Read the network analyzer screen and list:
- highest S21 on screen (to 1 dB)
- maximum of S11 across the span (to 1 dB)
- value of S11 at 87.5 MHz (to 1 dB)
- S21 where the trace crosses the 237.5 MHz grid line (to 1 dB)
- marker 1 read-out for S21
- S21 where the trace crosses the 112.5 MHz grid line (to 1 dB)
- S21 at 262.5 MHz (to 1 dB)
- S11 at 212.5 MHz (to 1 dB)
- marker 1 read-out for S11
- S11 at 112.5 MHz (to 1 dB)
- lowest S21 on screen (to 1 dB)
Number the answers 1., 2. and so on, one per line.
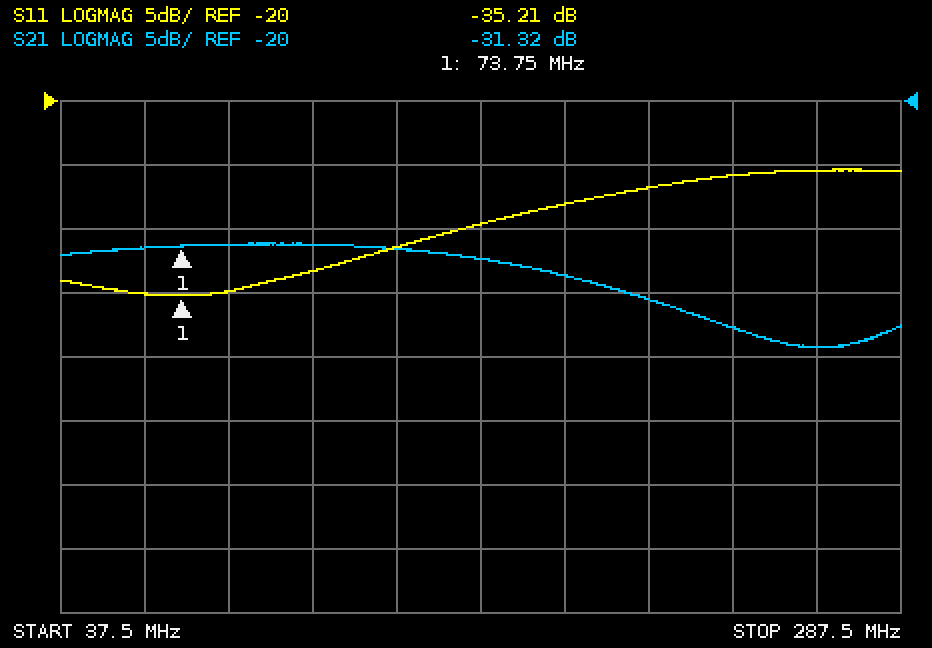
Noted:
1. -31 dB
2. -25 dB
3. -35 dB
4. -38 dB
5. -31.32 dB
6. -31 dB
7. -39 dB
8. -27 dB
9. -35.21 dB
10. -33 dB
11. -39 dB
